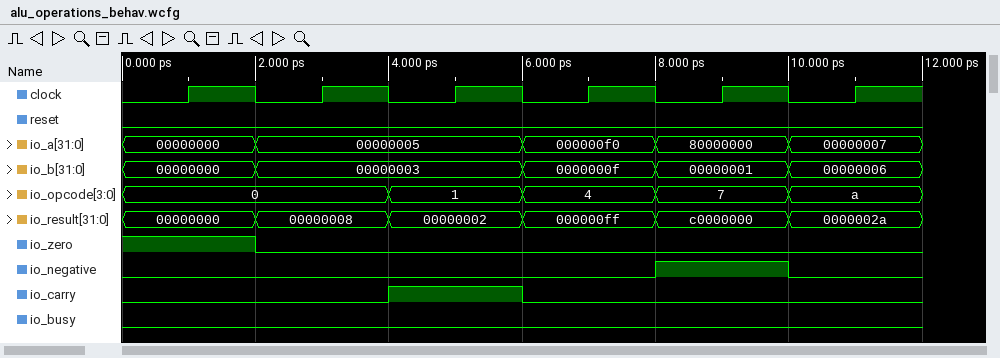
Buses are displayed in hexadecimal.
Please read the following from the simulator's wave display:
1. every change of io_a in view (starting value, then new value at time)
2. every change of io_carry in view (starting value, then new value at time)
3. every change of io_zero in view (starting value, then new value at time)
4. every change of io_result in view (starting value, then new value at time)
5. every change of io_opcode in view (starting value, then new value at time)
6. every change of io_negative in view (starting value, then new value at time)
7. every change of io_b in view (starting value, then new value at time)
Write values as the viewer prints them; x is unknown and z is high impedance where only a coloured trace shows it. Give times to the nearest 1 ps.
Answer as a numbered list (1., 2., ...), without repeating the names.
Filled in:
1. 00000000, 00000005 at 2 ps, 000000f0 at 6 ps, 80000000 at 8 ps, 00000007 at 10 ps
2. 0, 1 at 4 ps, 0 at 6 ps
3. 1, 0 at 2 ps
4. 00000000, 00000008 at 2 ps, 00000002 at 4 ps, 000000ff at 6 ps, c0000000 at 8 ps, 0000002a at 10 ps
5. 0, 1 at 4 ps, 4 at 6 ps, 7 at 8 ps, a at 10 ps
6. 0, 1 at 8 ps, 0 at 10 ps
7. 00000000, 00000003 at 2 ps, 0000000f at 6 ps, 00000001 at 8 ps, 00000006 at 10 ps
